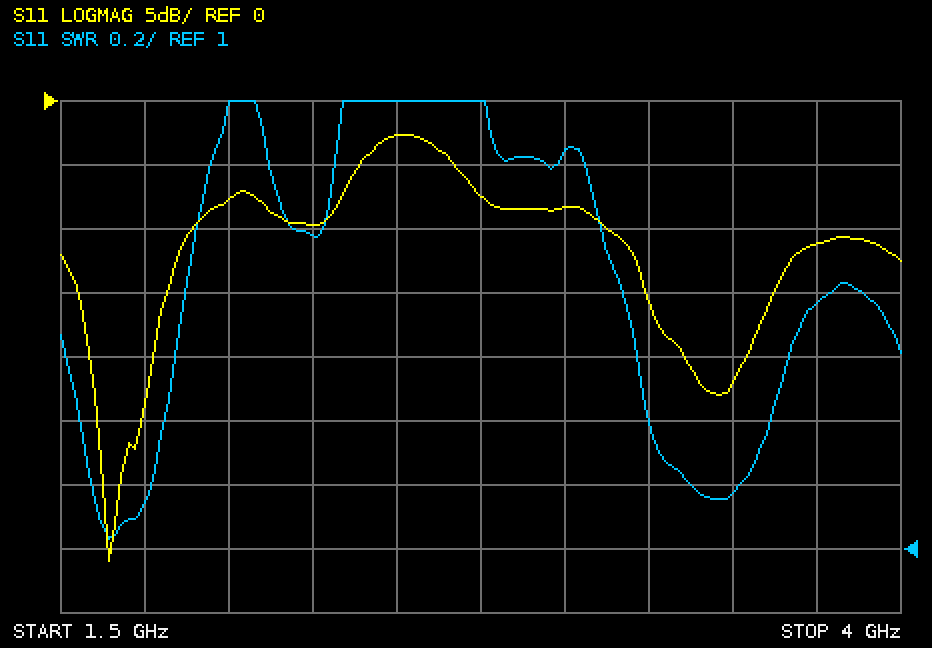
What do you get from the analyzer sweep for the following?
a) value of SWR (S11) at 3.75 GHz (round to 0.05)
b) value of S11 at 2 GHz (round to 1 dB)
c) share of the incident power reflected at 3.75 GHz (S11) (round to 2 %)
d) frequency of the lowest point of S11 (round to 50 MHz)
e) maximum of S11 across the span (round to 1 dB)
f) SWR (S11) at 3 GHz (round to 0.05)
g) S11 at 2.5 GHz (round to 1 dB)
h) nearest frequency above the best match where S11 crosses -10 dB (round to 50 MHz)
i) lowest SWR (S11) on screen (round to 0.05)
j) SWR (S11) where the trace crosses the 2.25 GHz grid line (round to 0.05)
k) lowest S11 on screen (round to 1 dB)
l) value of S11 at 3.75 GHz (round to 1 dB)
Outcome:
1.75
-8 dB
8 %
1.65 GHz
-3 dB
2.25
-3 dB
1.90 GHz
1.05
2.00
-36 dB
-11 dB
